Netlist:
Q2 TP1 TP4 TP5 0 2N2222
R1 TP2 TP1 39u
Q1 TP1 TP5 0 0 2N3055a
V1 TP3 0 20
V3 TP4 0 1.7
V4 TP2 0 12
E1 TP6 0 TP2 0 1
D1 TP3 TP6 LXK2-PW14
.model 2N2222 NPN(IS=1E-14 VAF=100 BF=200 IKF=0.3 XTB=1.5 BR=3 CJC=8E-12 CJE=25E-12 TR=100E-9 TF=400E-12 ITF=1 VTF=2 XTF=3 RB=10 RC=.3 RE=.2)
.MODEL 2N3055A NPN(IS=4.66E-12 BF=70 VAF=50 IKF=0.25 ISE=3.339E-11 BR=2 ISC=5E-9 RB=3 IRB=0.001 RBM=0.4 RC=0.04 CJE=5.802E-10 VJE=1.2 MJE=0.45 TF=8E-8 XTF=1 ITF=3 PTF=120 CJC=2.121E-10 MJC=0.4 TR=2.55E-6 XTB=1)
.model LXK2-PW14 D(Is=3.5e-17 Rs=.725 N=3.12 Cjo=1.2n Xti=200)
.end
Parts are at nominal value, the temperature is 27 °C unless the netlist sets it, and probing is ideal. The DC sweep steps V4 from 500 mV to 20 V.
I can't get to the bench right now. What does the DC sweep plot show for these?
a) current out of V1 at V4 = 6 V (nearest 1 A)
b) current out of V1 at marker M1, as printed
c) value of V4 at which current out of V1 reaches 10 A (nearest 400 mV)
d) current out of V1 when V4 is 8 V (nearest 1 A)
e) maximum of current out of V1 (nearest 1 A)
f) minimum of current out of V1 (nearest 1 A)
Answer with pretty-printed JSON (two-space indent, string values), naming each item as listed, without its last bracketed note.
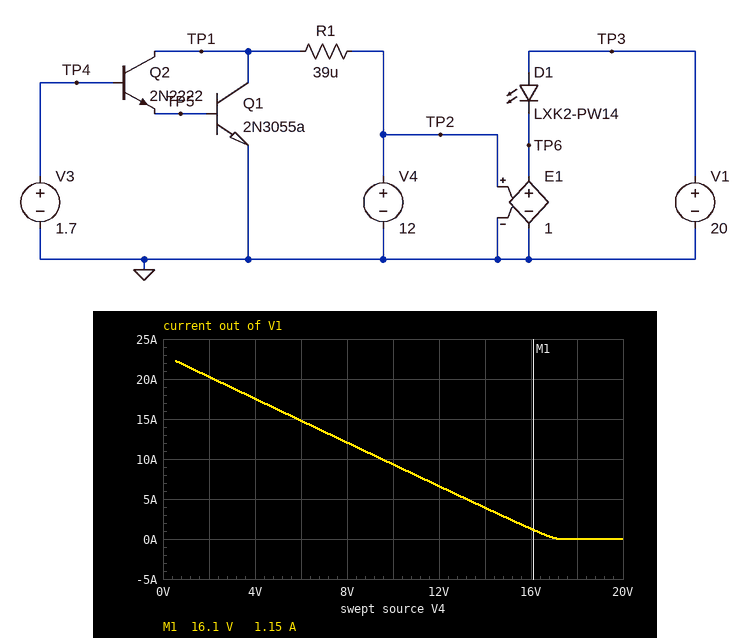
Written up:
{
  "current out of V1 at V4 = 6 V": "15 A",
  "current out of V1 at marker M1, as printed": "1.15 A",
  "value of V4 at which current out of V1 reaches 10 A": "9.6 V",
  "current out of V1 when V4 is 8 V": "12 A",
  "maximum of current out of V1": "22 A",
  "minimum of current out of V1": "0 A"
}
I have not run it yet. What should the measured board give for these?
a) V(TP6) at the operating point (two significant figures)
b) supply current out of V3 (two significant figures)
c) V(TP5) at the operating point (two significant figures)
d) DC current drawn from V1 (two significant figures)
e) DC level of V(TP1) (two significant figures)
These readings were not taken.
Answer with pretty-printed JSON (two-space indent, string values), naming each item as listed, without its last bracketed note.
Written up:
{
  "V(TP6) at the operating point": "12 V",
  "supply current out of V3": "1.4 mA",
  "V(TP5) at the operating point": "850 mV",
  "DC current drawn from V1": "6.6 A",
  "DC level of V(TP1)": "12 V"
}
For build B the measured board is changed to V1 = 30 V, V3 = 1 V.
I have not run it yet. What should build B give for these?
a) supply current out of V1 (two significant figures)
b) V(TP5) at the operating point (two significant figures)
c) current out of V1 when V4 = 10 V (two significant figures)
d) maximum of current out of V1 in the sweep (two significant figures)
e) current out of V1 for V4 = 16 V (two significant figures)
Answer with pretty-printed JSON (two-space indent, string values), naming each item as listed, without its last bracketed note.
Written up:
{
  "supply current out of V1": "20 A",
  "V(TP5) at the operating point": "470 mV",
  "current out of V1 when V4 = 10 V": "23 A",
  "maximum of current out of V1 in the sweep": "36 A",
  "current out of V1 for V4 = 16 V": "15 A"
}
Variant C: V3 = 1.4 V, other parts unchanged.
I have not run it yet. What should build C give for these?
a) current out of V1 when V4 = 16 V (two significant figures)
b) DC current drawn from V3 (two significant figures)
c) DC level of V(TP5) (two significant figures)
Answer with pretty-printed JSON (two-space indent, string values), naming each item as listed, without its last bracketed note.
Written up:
{
  "current out of V1 when V4 = 16 V": "1.3 A",
  "DC current drawn from V3": "56 µA",
  "DC level of V(TP5)": "680 mV"
}
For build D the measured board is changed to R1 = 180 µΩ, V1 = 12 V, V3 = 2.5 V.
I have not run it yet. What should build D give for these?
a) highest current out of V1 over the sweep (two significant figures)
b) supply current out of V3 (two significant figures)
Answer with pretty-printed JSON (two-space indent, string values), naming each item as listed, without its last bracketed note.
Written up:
{
  "highest current out of V1 over the sweep": "11 A",
  "supply current out of V3": "18 mA"
}
